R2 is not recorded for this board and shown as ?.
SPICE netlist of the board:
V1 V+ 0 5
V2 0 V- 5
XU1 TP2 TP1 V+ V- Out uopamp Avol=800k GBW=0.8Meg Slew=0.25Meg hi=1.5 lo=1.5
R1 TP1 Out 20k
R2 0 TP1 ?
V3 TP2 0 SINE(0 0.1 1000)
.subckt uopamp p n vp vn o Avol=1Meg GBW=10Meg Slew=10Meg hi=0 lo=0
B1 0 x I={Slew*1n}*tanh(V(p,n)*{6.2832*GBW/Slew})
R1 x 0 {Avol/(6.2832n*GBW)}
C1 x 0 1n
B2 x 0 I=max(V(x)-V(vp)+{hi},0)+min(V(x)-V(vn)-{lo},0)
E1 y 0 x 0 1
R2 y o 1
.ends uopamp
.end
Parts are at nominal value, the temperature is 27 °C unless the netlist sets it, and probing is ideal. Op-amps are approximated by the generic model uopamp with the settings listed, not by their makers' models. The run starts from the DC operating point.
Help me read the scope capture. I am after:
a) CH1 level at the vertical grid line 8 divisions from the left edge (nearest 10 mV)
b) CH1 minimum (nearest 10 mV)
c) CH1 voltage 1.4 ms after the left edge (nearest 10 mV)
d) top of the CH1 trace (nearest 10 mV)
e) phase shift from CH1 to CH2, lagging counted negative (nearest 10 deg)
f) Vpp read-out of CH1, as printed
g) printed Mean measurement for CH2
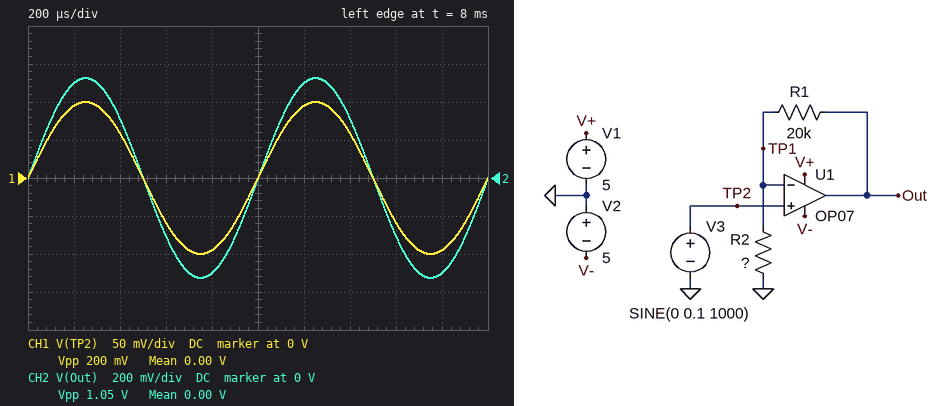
-60 mV
-100 mV
60 mV
100 mV
0 deg
200 mV
0.00 V
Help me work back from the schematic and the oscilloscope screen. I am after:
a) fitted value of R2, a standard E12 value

4.7 kΩ
